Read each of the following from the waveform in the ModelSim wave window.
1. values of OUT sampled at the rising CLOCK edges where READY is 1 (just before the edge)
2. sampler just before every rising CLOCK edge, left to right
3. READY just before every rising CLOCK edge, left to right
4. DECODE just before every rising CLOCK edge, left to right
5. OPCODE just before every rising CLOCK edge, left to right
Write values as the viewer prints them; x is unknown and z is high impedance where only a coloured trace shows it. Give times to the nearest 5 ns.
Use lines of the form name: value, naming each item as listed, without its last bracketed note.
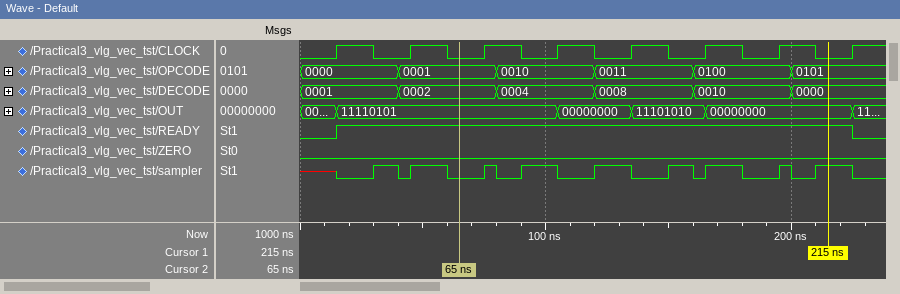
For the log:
values of OUT sampled at the rising CLOCK edges where READY is 1: 11110101, 11110101, 11110101, 00000000, 11101010, 00000000, 00000000
sampler just before every rising CLOCK edge, left to right: x 0 0 1 1 0 0 1
READY just before every rising CLOCK edge, left to right: 0 1 1 1 1 1 1 1
DECODE just before every rising CLOCK edge, left to right: 0001, 0002, 0002, 0004, 0008, 0010, 0010, 0000
OPCODE just before every rising CLOCK edge, left to right: 0000, 0001, 0001, 0010, 0011, 0100, 0100, 0101
